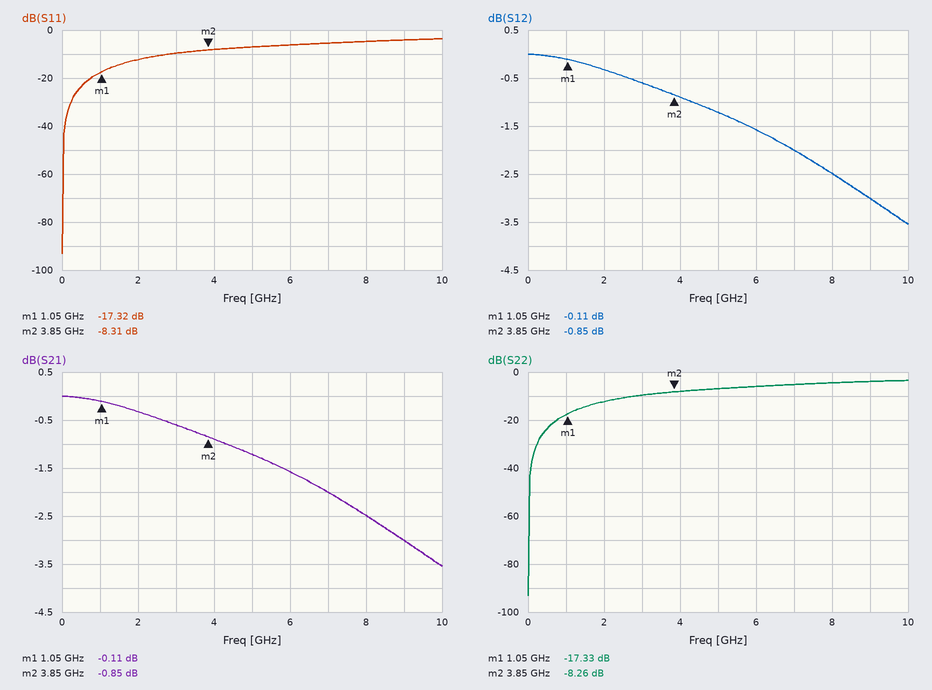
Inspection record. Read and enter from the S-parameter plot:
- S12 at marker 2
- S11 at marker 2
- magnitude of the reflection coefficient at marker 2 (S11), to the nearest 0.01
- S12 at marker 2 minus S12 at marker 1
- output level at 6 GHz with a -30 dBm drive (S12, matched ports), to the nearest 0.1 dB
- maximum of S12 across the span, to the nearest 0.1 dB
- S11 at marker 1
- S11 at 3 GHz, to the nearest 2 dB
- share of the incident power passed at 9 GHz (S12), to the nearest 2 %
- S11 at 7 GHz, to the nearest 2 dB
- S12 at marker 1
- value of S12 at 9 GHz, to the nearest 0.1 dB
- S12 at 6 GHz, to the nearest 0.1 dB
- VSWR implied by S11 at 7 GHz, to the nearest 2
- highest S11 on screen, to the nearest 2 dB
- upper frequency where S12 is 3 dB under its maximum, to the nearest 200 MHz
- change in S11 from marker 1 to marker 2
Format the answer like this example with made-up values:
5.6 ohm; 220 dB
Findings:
-0.85 dB; -8.31 dB; 0.38; -0.74 dB; -31.6 dBm; 0.0 dB; -17.32 dB; -10 dB; 50 %; -6 dB; -0.11 dB; -3.0 dB; -1.6 dB; 4; -4 dB; 9.0 GHz; 9.01 dB
